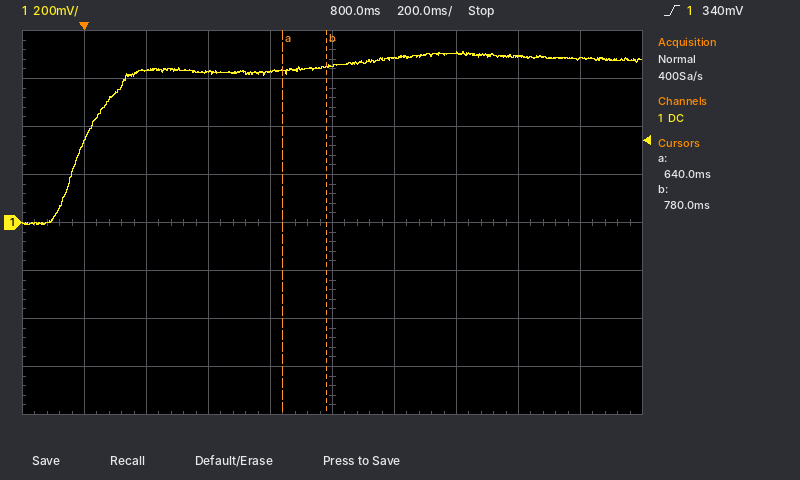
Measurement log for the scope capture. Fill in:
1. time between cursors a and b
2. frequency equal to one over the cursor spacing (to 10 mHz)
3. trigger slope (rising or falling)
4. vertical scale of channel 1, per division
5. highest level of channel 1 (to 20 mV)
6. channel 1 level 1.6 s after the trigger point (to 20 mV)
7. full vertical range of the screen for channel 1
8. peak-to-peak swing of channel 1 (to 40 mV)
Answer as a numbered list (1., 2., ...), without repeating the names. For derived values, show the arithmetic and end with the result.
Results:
1. 780 ms − (640 ms) = 140 ms
2. 1 / 140 ms ≈ 7.14 Hz
3. rising
4. 200 mV
5. 720 mV
6. 680 mV
7. 1.6 V
8. 720 mV
